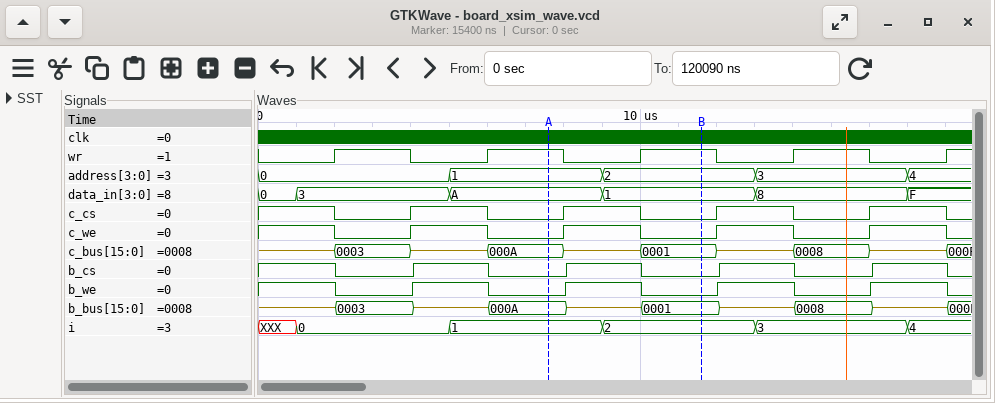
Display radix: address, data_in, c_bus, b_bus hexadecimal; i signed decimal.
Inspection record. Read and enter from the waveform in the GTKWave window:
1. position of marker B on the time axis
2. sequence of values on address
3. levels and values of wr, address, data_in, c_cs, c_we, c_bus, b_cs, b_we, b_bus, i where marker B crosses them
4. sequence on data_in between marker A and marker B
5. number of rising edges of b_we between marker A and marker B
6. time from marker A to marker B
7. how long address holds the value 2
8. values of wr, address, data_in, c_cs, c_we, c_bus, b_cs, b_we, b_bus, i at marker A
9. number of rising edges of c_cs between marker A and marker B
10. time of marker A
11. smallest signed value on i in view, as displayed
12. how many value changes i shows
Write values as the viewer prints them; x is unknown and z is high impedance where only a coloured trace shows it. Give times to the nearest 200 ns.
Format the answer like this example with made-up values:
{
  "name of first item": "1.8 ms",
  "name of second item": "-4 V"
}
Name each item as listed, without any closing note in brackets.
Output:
{
  "position of marker B on the time axis": "11600 ns",
  "sequence of values on address": "0, 1, 2, 3, 4",
  "levels and values of wr, address, data_in, c_cs, c_we, c_bus, b_cs, b_we, b_bus, i where marker B crosses them": "wr=1, address=2, data_in=1, c_cs=0, c_we=0, c_bus=0001, b_cs=0, b_we=0, b_bus=0001, i=2",
  "sequence on data_in between marker A and marker B": "A, 1",
  "number of rising edges of b_we between marker A and marker B": "1",
  "time from marker A to marker B": "4000 ns",
  "how long address holds the value 2": "4000 ns",
  "values of wr, address, data_in, c_cs, c_we, c_bus, b_cs, b_we, b_bus, i at marker A": "wr=1, address=1, data_in=A, c_cs=0, c_we=0, c_bus=000A, b_cs=0, b_we=0, b_bus=000A, i=1",
  "number of rising edges of c_cs between marker A and marker B": "1",
  "time of marker A": "7600 ns",
  "smallest signed value on i in view, as displayed": "0",
  "how many value changes i shows": "5"
}
